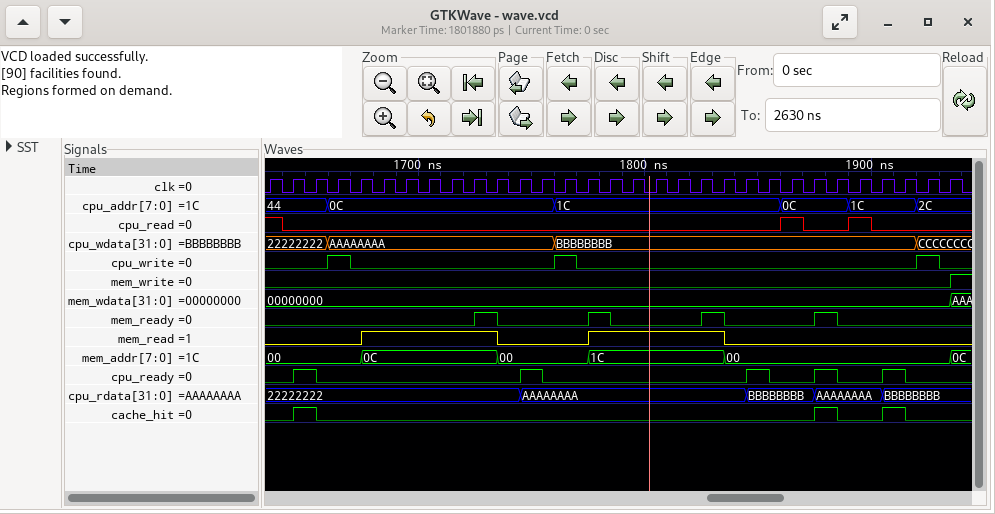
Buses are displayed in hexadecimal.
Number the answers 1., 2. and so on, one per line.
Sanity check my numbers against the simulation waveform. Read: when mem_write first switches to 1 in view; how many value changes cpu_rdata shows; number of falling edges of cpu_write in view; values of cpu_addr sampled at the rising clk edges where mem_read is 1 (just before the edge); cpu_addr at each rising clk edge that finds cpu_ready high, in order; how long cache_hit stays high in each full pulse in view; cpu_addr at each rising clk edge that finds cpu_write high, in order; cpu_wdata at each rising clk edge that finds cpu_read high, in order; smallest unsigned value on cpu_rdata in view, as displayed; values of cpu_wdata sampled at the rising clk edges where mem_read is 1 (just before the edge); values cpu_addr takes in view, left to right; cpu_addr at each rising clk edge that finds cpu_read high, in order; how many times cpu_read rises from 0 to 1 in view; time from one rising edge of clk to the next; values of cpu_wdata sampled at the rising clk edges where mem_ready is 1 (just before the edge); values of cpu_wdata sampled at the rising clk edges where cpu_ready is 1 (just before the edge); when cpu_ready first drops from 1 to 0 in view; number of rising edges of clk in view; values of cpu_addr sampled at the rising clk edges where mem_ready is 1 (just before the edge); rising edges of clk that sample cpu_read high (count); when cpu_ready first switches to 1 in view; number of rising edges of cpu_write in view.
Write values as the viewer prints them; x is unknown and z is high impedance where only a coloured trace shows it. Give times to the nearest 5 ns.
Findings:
1. 1935 ns
2. 4
3. 3
4. 0C, 0C, 0C, 0C, 0C, 0C, 1C, 1C, 1C, 1C, 1C, 1C
5. 44, 0C, 1C, 0C, 1C
6. 10 ns, 10 ns, 10 ns
7. 0C, 1C, 2C
8. 22222222, BBBBBBBB, BBBBBBBB
9. 22222222
10. AAAAAAAA, AAAAAAAA, AAAAAAAA, AAAAAAAA, AAAAAAAA, AAAAAAAA, BBBBBBBB, BBBBBBBB, BBBBBBBB, BBBBBBBB, BBBBBBBB, BBBBBBBB
11. 44, 0C, 1C, 0C, 1C, 2C
12. 44, 0C, 1C
13. 2
14. 10 ns
15. AAAAAAAA, BBBBBBBB, BBBBBBBB, BBBBBBBB
16. 22222222, AAAAAAAA, BBBBBBBB, BBBBBBBB, BBBBBBBB
17. 1655 ns
18. 31
19. 0C, 1C, 1C, 0C
20. 3
21. 1645 ns
22. 3
